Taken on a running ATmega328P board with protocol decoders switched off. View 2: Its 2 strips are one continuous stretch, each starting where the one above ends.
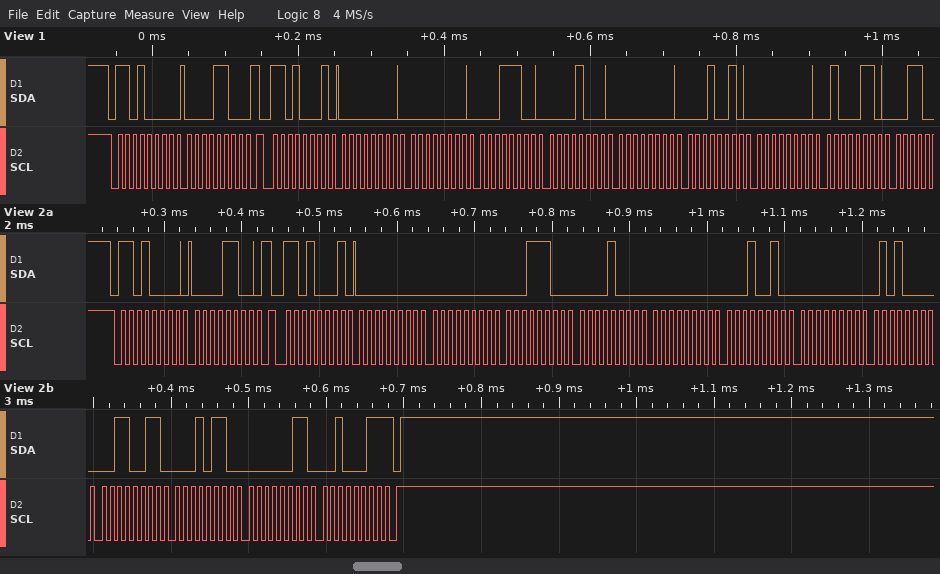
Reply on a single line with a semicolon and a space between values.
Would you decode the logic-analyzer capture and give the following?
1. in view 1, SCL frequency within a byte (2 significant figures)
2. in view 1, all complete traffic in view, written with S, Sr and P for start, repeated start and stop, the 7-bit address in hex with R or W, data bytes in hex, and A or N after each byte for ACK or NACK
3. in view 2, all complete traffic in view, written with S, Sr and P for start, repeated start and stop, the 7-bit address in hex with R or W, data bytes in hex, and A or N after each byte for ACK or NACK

100 kHz; S 68W A 0C A Sr 68R A 00 A 00 A 1C A 08 A 00 A 12 A 00 A 46 A; S 68W A 0C A Sr 68R A 00 A 00 A 1C A 08 A 00 A 12 A 00 A 50 A 33 A 16 A 03 A 23 N P
